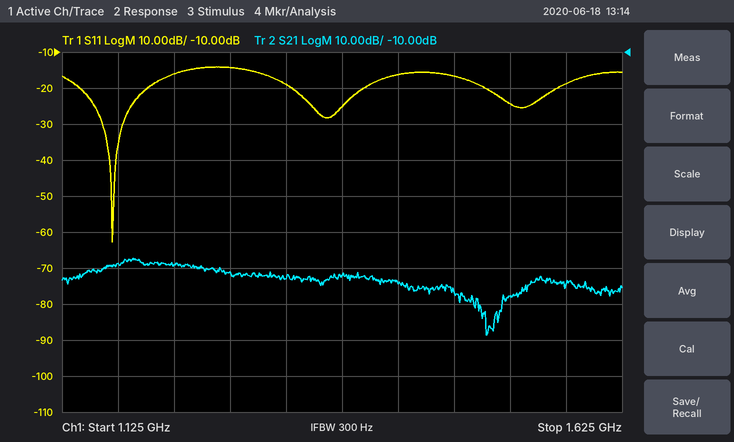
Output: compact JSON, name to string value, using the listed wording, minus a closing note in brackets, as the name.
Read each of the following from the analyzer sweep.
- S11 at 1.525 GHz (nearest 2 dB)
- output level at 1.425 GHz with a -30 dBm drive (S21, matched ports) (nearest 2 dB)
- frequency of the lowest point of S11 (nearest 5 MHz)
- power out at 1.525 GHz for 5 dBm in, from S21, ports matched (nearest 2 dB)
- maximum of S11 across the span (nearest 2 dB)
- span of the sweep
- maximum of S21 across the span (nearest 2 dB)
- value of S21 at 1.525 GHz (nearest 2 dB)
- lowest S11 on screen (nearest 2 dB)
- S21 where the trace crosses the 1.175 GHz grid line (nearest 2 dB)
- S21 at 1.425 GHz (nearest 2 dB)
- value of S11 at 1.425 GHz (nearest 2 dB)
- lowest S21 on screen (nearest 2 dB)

{"S11 at 1.525 GHz": "-24 dB", "output level at 1.425 GHz with a -30 dBm drive (S21, matched ports)": "-104 dBm", "frequency of the lowest point of S11": "1.170 GHz", "power out at 1.525 GHz for 5 dBm in, from S21, ports matched": "-72 dBm", "maximum of S11 across the span": "-14 dB", "span of the sweep": "500 MHz", "maximum of S21 across the span": "-68 dB", "value of S21 at 1.525 GHz": "-78 dB", "lowest S11 on screen": "-62 dB", "S21 where the trace crosses the 1.175 GHz grid line": "-68 dB", "S21 at 1.425 GHz": "-74 dB", "value of S11 at 1.425 GHz": "-16 dB", "lowest S21 on screen": "-88 dB"}
